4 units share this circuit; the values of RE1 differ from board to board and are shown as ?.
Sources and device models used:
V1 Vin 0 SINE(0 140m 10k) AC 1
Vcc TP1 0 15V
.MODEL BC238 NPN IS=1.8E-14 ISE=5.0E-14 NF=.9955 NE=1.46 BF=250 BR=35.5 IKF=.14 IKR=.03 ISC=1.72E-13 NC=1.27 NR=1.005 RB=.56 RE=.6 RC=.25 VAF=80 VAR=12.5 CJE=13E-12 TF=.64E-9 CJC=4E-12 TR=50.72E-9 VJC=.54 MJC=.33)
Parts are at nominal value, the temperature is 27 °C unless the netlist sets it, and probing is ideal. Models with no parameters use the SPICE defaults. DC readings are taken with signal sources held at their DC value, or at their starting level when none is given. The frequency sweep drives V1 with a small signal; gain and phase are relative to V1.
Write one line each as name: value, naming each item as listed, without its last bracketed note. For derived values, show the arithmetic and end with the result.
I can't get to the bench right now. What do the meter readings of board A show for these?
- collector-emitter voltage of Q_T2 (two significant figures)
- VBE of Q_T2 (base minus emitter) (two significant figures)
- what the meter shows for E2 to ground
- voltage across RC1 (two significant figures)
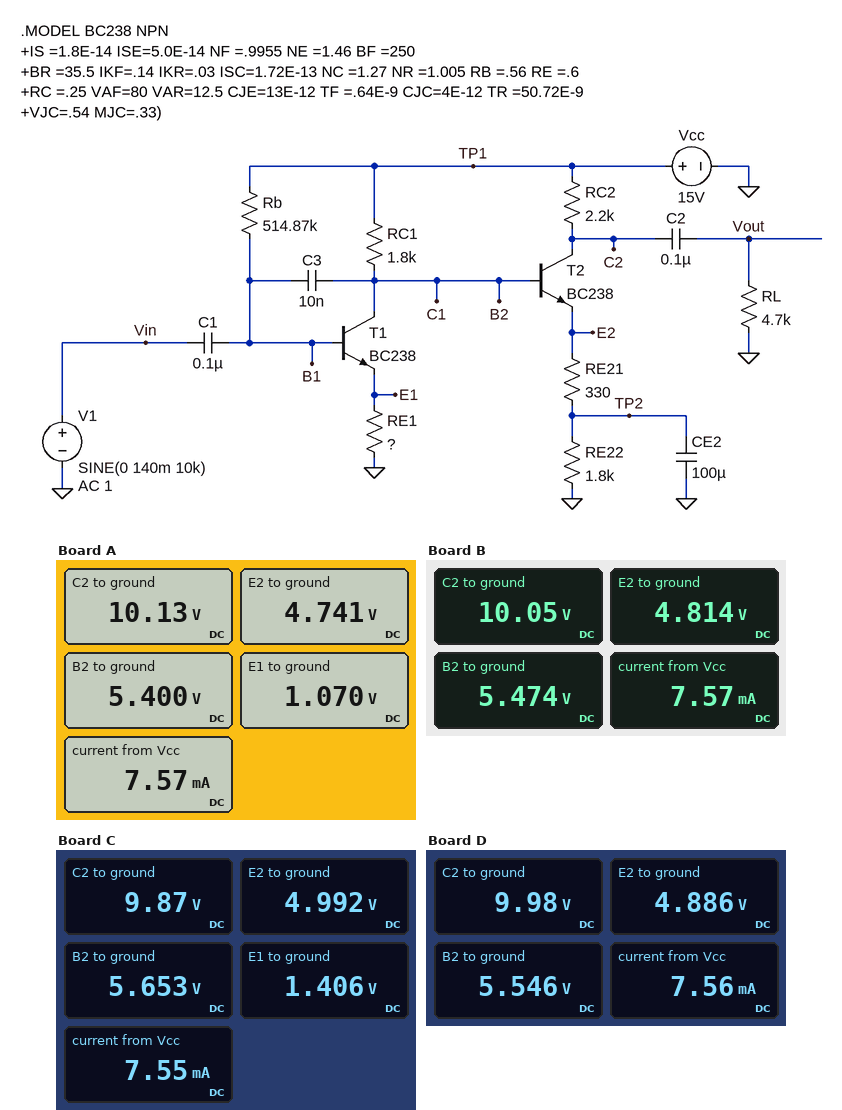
collector-emitter voltage of Q_T2: 10.13 V - 4.741 V = 5.4 V
VBE of Q_T2 (base minus emitter): 5.4 V - 4.741 V = 660 mV
what the meter shows for E2 to ground: 4.741 V
voltage across RC1: 15 V - 5.4 V = 9.6 V
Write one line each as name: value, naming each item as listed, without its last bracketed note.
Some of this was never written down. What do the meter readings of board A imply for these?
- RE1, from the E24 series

RE1, from the E24 series: 200 Ω
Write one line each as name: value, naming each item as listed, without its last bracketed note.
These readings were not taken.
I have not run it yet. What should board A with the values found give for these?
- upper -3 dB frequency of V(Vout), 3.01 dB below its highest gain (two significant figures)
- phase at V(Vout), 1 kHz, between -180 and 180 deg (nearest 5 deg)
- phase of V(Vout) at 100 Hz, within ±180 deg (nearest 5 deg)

upper -3 dB frequency of V(Vout), 3.01 dB below its highest gain: 19 kHz
phase at V(Vout), 1 kHz, between -180 and 180 deg: 10 deg
phase of V(Vout) at 100 Hz, within ±180 deg: 80 deg
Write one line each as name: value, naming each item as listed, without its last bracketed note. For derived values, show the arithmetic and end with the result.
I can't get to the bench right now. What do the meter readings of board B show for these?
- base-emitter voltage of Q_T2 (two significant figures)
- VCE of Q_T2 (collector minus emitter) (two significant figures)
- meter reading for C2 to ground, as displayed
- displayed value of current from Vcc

base-emitter voltage of Q_T2: 5.474 V - 4.814 V = 660 mV
VCE of Q_T2 (collector minus emitter): 10.05 V - 4.814 V = 5.2 V
meter reading for C2 to ground, as displayed: 10.05 V
displayed value of current from Vcc: 7.57 mA
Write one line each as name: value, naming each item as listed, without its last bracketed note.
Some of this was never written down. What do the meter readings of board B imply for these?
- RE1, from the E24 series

RE1, from the E24 series: 220 Ω
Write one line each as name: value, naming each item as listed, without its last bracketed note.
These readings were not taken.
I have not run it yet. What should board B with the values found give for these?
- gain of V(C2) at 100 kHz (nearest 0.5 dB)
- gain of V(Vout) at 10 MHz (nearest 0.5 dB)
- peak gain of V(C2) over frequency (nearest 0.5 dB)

gain of V(C2) at 100 kHz: 14.5 dB
gain of V(Vout) at 10 MHz: 12.5 dB
peak gain of V(C2) over frequency: 28.0 dB
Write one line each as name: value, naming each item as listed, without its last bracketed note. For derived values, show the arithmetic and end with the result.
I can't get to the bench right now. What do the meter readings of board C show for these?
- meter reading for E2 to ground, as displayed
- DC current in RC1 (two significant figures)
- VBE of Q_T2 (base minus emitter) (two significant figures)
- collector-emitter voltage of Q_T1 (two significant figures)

meter reading for E2 to ground, as displayed: 4.992 V
DC current in RC1: (15 V - 5.653 V) / 1.8 kΩ = 5.2 mA
VBE of Q_T2 (base minus emitter): 5.653 V - 4.992 V = 660 mV
collector-emitter voltage of Q_T1: 5.653 V - 1.406 V = 4.2 V
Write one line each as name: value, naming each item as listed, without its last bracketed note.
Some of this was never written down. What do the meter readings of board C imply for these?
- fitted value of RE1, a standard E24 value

fitted value of RE1, a standard E24 value: 270 Ω
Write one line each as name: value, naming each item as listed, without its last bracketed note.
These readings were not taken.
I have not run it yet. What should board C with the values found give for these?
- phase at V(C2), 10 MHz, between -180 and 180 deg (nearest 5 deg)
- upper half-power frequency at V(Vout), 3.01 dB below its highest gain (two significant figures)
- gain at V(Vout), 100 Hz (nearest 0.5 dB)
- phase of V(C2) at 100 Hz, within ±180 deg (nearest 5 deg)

phase at V(C2), 10 MHz, between -180 and 180 deg: 165 deg
upper half-power frequency at V(Vout), 3.01 dB below its highest gain: 18 kHz
gain at V(Vout), 100 Hz: 16.0 dB
phase of V(C2) at 100 Hz, within ±180 deg: 5 deg
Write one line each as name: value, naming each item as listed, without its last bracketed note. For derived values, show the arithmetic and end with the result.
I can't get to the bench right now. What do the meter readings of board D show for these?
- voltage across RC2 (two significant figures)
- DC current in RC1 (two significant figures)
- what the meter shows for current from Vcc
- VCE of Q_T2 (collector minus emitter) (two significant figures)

voltage across RC2: 15 V - 9.98 V = 5.0 V
DC current in RC1: (15 V - 5.546 V) / 1.8 kΩ = 5.3 mA
what the meter shows for current from Vcc: 7.56 mA
VCE of Q_T2 (collector minus emitter): 9.98 V - 4.886 V = 5.1 V
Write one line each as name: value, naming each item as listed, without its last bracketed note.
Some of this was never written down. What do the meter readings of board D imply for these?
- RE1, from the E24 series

RE1, from the E24 series: 240 Ω
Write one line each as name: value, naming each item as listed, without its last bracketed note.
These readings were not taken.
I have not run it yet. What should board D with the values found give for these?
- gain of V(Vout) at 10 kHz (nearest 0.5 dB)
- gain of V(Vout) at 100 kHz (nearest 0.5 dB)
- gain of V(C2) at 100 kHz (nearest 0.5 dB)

gain of V(Vout) at 10 kHz: 23.5 dB
gain of V(Vout) at 100 kHz: 14.0 dB
gain of V(C2) at 100 kHz: 14.0 dB
